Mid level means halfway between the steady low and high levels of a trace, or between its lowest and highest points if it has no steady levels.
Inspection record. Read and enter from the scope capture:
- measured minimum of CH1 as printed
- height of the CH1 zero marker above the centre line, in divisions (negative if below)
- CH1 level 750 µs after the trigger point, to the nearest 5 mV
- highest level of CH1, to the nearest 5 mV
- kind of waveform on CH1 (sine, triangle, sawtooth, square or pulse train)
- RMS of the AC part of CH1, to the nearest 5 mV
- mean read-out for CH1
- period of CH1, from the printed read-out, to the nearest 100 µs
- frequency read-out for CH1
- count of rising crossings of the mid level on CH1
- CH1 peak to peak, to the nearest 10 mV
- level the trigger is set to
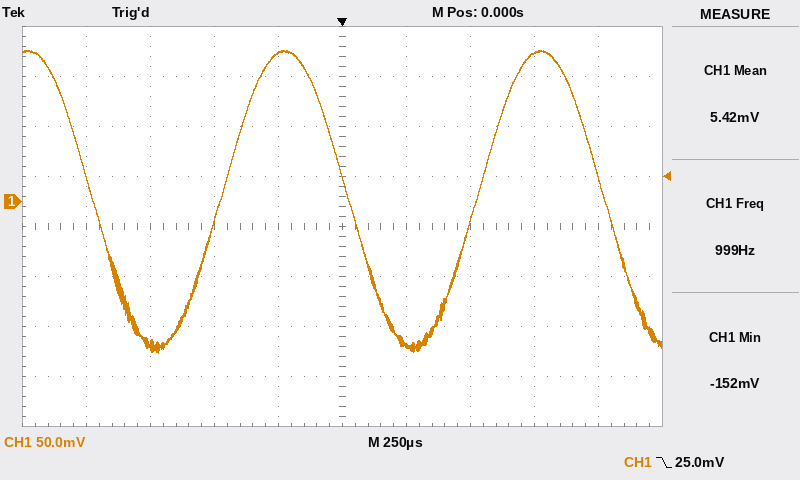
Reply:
-152 mV
+0.5 div
150 mV
150 mV
sine
105 mV
5.42 mV
1.0 ms
999 Hz
2
300 mV
25.0 mV
